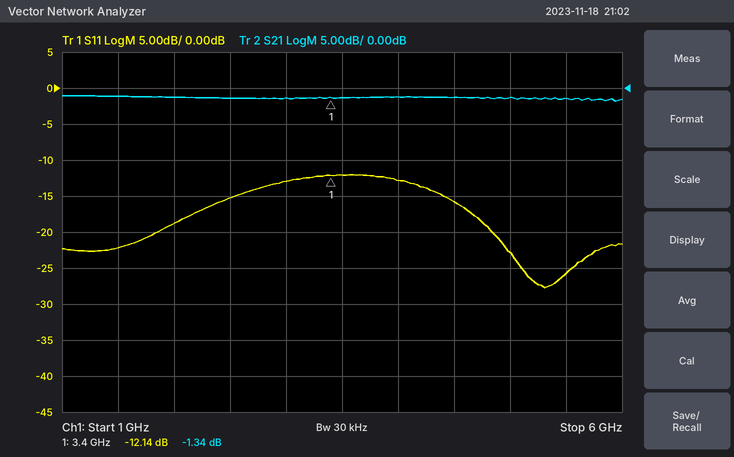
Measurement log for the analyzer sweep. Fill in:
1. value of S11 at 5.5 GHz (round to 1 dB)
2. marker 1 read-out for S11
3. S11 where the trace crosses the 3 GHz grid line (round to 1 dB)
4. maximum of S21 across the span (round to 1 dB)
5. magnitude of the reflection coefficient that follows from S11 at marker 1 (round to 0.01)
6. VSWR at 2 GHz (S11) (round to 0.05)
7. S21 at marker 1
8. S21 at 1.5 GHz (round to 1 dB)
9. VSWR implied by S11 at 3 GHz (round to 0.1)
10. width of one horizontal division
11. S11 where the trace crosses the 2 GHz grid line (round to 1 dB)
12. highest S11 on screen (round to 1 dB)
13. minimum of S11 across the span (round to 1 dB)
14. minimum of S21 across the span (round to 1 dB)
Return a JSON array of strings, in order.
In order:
["-26 dB", "-12.14 dB", "-13 dB", "-1 dB", "0.25", "1.25", "-1.34 dB", "-1 dB", "1.6", "500 MHz", "-19 dB", "-12 dB", "-28 dB", "-2 dB"]
